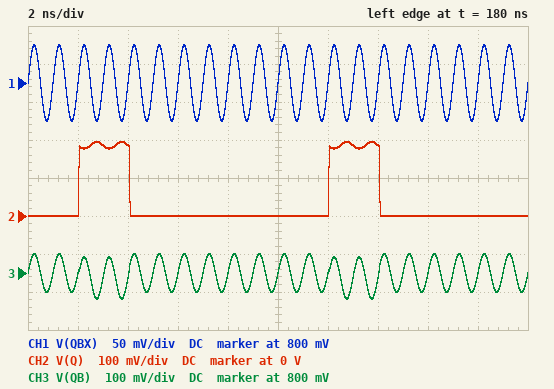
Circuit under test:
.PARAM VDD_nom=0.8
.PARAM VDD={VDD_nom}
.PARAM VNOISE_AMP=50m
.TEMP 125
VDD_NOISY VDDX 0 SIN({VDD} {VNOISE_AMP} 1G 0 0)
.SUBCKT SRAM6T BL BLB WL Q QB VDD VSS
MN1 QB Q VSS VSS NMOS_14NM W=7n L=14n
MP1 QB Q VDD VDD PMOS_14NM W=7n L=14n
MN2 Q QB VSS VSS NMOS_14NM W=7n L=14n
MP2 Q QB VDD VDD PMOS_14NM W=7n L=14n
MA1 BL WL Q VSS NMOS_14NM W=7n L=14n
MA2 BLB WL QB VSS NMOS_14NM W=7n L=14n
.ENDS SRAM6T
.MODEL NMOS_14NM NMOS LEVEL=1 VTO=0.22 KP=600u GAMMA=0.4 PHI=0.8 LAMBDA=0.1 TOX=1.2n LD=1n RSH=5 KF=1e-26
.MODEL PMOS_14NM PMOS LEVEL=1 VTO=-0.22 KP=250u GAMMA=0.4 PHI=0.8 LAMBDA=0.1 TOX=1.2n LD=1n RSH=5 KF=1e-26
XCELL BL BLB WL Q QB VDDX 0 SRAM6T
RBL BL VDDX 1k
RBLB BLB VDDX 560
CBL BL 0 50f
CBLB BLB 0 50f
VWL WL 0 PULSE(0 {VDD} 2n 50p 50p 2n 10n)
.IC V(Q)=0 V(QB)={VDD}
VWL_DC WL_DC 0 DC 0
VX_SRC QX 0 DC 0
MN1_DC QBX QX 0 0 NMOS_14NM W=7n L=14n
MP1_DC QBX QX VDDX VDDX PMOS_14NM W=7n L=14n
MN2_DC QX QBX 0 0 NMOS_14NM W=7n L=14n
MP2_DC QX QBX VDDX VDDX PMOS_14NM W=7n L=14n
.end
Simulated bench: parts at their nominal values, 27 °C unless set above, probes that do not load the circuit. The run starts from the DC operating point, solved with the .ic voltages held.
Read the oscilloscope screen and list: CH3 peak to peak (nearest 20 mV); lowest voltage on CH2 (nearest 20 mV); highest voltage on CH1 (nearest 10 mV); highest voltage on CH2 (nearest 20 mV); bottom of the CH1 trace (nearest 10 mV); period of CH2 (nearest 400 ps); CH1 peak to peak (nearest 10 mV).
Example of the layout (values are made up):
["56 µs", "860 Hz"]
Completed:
["120 mV", "0 V", "850 mV", "200 mV", "750 mV", "10.0 ns", "100 mV"]
